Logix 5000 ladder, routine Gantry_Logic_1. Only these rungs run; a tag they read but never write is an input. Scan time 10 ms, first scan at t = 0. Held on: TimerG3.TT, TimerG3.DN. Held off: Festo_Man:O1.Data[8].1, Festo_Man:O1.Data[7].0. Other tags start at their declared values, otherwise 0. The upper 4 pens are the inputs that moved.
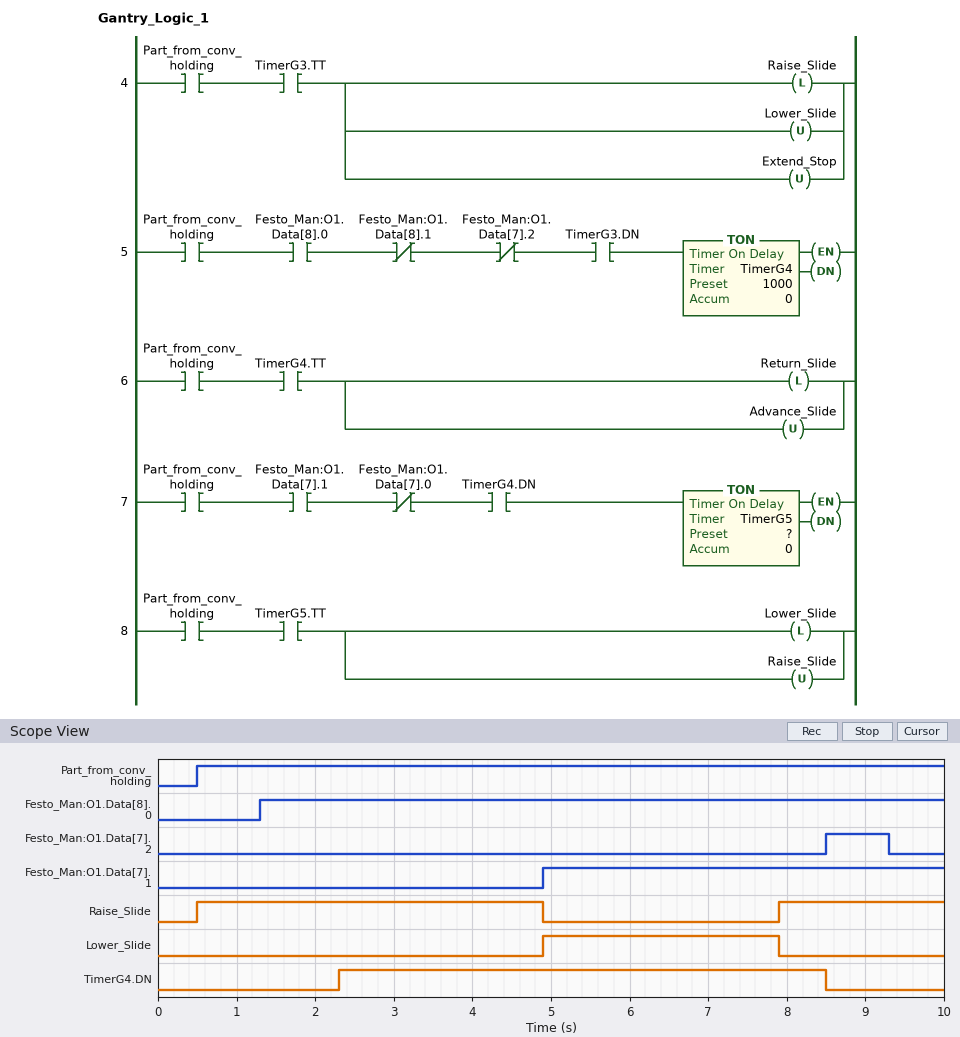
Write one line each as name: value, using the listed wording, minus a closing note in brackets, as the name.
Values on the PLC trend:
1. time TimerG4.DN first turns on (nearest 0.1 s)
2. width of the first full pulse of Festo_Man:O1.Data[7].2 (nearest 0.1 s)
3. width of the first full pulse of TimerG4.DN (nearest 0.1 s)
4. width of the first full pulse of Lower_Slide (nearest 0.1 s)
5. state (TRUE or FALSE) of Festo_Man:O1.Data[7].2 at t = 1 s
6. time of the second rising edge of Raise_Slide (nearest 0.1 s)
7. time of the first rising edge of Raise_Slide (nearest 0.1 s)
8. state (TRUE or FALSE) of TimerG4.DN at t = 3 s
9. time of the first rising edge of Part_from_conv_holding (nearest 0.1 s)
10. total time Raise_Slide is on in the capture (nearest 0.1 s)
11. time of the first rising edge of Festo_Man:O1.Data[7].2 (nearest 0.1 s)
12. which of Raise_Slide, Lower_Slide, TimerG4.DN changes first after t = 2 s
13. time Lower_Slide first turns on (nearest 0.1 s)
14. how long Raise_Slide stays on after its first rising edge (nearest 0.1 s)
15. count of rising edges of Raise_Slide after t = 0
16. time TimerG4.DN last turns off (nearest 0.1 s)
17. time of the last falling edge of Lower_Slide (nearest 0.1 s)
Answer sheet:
time TimerG4.DN first turns on: 2.3 s
width of the first full pulse of Festo_Man:O1.Data[7].2: 0.8 s
width of the first full pulse of TimerG4.DN: 6.2 s
width of the first full pulse of Lower_Slide: 3.0 s
state (TRUE or FALSE) of Festo_Man:O1.Data[7].2 at t = 1 s: FALSE
time of the second rising edge of Raise_Slide: 7.9 s
time of the first rising edge of Raise_Slide: 0.5 s
state (TRUE or FALSE) of TimerG4.DN at t = 3 s: TRUE
time of the first rising edge of Part_from_conv_holding: 0.5 s
total time Raise_Slide is on in the capture: 6.5 s
time of the first rising edge of Festo_Man:O1.Data[7].2: 8.5 s
which of Raise_Slide, Lower_Slide, TimerG4.DN changes first after t = 2 s: TimerG4.DN
time Lower_Slide first turns on: 4.9 s
how long Raise_Slide stays on after its first rising edge: 4.4 s
count of rising edges of Raise_Slide after t = 0: 2
time TimerG4.DN last turns off: 8.5 s
time of the last falling edge of Lower_Slide: 7.9 s
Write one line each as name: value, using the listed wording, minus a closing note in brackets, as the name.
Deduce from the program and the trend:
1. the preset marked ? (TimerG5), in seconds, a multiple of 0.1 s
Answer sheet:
the preset marked ? (TimerG5), in seconds, a multiple of 0.1 s: 3.0 s
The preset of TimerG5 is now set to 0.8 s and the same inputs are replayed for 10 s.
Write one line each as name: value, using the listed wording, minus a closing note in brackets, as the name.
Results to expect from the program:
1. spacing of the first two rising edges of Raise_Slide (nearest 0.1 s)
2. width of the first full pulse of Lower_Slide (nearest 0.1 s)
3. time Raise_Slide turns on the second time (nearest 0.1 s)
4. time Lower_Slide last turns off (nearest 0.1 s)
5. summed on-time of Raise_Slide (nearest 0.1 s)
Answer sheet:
spacing of the first two rising edges of Raise_Slide: 5.2 s
width of the first full pulse of Lower_Slide: 0.8 s
time Raise_Slide turns on the second time: 5.7 s
time Lower_Slide last turns off: 5.7 s
summed on-time of Raise_Slide: 8.7 s
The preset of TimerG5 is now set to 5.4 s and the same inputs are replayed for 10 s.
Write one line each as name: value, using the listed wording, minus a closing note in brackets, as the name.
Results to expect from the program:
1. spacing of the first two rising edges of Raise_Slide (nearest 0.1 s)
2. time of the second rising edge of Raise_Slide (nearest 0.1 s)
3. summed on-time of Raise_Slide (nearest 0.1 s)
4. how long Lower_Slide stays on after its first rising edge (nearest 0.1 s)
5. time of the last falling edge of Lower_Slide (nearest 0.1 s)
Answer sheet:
spacing of the first two rising edges of Raise_Slide: 8.0 s
time of the second rising edge of Raise_Slide: 8.5 s
summed on-time of Raise_Slide: 5.9 s
how long Lower_Slide stays on after its first rising edge: 3.6 s
time of the last falling edge of Lower_Slide: 8.5 s
